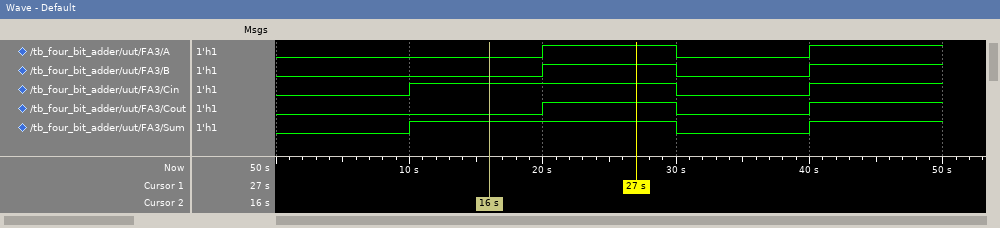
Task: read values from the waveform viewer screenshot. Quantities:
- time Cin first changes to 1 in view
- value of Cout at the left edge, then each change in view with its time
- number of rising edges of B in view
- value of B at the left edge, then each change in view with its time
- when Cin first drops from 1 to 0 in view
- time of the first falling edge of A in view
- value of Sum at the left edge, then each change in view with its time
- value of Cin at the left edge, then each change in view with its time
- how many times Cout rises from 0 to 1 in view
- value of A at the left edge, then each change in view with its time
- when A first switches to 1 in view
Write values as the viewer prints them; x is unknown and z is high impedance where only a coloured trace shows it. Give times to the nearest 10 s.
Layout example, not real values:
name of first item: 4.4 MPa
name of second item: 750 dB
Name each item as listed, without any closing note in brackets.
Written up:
time Cin first changes to 1 in view: 10 s
value of Cout at the left edge, then each change in view with its time: 0, 1 at 20 s, 0 at 30 s, 1 at 40 s
number of rising edges of B in view: 2
value of B at the left edge, then each change in view with its time: 0, 1 at 20 s, 0 at 30 s, 1 at 40 s
when Cin first drops from 1 to 0 in view: 30 s
time of the first falling edge of A in view: 30 s
value of Sum at the left edge, then each change in view with its time: 0, 1 at 10 s, 0 at 30 s, 1 at 40 s
value of Cin at the left edge, then each change in view with its time: 0, 1 at 10 s, 0 at 30 s, 1 at 40 s
how many times Cout rises from 0 to 1 in view: 2
value of A at the left edge, then each change in view with its time: 0, 1 at 20 s, 0 at 30 s, 1 at 40 s
when A first switches to 1 in view: 20 s
